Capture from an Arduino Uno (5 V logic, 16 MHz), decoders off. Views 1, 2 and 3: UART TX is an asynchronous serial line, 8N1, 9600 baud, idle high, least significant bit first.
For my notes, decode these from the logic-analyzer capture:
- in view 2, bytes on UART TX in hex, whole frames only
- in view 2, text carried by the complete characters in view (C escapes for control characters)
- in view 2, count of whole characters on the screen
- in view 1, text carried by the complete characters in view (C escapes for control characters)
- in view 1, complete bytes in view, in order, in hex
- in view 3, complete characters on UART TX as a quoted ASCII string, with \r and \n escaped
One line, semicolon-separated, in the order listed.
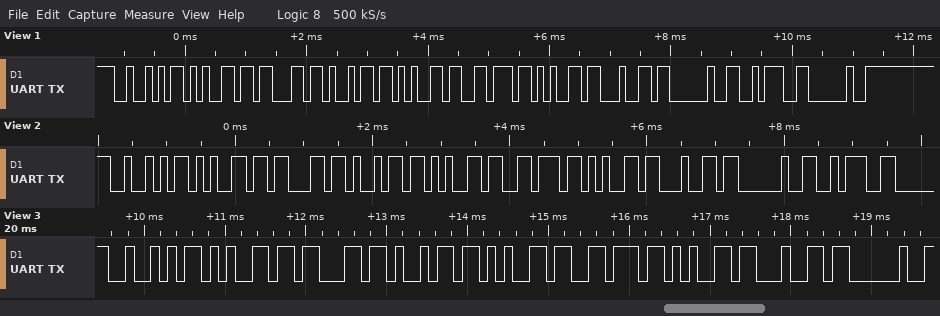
52 65 63 69 65 76 65 64 20 3A; "Recieved :"; 10; "Recieved : "; 52 65 63 69 65 76 65 64 20 3A 20; "Recieved "
